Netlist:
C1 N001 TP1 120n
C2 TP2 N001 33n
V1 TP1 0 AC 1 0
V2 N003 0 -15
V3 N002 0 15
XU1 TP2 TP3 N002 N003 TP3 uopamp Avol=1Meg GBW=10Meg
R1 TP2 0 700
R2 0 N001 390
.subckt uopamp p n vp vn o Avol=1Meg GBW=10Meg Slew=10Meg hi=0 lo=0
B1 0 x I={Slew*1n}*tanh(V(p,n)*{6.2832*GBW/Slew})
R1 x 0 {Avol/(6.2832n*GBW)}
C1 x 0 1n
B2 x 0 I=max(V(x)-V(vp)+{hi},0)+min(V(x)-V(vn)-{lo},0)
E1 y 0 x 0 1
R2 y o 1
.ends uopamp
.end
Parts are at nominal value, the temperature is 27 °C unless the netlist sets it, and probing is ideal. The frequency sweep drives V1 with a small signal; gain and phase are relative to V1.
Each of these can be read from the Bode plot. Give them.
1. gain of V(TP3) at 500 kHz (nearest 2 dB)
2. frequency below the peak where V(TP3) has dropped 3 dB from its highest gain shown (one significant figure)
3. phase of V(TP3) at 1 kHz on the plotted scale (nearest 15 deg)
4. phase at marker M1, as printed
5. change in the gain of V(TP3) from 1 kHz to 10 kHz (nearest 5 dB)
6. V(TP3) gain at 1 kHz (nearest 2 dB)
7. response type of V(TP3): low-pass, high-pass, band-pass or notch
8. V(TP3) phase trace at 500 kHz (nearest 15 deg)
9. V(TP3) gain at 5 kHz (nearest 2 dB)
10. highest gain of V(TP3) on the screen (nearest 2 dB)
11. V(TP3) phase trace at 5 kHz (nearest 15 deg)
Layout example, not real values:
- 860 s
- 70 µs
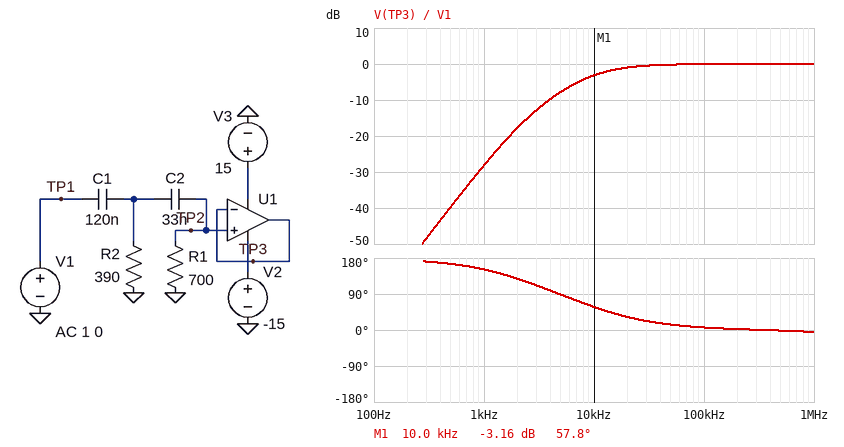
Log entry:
- 0 dB
- 10 kHz
- 150 deg
- 57.8 deg
- 25 dB
- -28 dB
- high-pass
- 0 deg
- -8 dB
- 0 dB
- 90 deg
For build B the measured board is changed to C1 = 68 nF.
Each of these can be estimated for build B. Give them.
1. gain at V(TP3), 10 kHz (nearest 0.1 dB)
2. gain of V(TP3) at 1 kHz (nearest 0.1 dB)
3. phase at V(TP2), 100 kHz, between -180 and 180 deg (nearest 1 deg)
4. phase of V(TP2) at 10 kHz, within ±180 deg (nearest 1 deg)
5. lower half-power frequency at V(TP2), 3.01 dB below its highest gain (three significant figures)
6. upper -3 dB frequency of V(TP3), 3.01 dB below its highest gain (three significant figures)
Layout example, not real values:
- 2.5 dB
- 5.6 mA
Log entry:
- -4.7 dB
- -32.8 dB
- 9 deg
- 70 deg
- 13.8 kHz
- 10.0 MHz
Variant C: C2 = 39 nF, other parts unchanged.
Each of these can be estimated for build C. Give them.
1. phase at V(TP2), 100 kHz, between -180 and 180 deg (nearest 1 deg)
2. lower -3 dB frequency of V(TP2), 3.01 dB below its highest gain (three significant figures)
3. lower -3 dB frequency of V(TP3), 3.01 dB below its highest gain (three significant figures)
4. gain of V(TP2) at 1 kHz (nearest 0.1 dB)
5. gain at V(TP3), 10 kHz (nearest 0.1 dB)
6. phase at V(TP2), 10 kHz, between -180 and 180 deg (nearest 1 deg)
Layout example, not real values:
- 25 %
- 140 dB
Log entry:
- 6 deg
- 9.41 kHz
- 9.39 kHz
- -26.8 dB
- -2.7 dB
- 54 deg
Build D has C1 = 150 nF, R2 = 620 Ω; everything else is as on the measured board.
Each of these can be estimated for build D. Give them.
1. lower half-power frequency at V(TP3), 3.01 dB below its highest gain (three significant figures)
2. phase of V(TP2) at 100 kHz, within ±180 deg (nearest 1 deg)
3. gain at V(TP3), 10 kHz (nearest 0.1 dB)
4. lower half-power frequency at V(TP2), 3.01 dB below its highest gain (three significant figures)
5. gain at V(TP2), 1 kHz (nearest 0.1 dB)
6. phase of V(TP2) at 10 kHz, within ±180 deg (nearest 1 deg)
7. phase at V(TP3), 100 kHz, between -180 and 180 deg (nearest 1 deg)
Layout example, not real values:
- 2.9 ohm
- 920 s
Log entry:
- 8.96 kHz
- 6 deg
- -2.6 dB
- 8.97 kHz
- -23.4 dB
- 49 deg
- 5 deg
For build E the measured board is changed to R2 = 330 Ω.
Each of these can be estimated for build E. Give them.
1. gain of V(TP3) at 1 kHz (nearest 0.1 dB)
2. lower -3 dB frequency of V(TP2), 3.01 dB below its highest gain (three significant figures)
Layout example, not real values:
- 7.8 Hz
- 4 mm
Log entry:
- -29.4 dB
- 10.7 kHz
